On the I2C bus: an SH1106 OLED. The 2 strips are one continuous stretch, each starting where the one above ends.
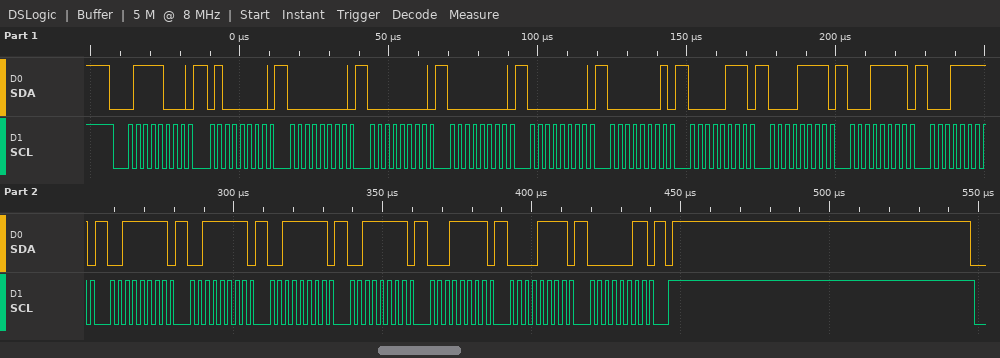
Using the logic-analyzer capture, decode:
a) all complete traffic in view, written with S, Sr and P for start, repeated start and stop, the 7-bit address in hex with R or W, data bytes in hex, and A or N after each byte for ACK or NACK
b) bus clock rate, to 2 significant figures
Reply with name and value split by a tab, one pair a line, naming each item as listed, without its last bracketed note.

all complete traffic in view, written with S, Sr and P for start, repeated start and stop, the 7-bit address in hex with R or W, data bytes in hex, and A or N after each byte for ACK or NACK	S 3CW A 40 A 00 A 00 A 00 A 00 A 01 A 07 A 0F A 1F A 1F A 3F A 3F A 3F A 3F A 1F A 0F A 03 A P
bus clock rate, to 2 significant figures	400 kHz
